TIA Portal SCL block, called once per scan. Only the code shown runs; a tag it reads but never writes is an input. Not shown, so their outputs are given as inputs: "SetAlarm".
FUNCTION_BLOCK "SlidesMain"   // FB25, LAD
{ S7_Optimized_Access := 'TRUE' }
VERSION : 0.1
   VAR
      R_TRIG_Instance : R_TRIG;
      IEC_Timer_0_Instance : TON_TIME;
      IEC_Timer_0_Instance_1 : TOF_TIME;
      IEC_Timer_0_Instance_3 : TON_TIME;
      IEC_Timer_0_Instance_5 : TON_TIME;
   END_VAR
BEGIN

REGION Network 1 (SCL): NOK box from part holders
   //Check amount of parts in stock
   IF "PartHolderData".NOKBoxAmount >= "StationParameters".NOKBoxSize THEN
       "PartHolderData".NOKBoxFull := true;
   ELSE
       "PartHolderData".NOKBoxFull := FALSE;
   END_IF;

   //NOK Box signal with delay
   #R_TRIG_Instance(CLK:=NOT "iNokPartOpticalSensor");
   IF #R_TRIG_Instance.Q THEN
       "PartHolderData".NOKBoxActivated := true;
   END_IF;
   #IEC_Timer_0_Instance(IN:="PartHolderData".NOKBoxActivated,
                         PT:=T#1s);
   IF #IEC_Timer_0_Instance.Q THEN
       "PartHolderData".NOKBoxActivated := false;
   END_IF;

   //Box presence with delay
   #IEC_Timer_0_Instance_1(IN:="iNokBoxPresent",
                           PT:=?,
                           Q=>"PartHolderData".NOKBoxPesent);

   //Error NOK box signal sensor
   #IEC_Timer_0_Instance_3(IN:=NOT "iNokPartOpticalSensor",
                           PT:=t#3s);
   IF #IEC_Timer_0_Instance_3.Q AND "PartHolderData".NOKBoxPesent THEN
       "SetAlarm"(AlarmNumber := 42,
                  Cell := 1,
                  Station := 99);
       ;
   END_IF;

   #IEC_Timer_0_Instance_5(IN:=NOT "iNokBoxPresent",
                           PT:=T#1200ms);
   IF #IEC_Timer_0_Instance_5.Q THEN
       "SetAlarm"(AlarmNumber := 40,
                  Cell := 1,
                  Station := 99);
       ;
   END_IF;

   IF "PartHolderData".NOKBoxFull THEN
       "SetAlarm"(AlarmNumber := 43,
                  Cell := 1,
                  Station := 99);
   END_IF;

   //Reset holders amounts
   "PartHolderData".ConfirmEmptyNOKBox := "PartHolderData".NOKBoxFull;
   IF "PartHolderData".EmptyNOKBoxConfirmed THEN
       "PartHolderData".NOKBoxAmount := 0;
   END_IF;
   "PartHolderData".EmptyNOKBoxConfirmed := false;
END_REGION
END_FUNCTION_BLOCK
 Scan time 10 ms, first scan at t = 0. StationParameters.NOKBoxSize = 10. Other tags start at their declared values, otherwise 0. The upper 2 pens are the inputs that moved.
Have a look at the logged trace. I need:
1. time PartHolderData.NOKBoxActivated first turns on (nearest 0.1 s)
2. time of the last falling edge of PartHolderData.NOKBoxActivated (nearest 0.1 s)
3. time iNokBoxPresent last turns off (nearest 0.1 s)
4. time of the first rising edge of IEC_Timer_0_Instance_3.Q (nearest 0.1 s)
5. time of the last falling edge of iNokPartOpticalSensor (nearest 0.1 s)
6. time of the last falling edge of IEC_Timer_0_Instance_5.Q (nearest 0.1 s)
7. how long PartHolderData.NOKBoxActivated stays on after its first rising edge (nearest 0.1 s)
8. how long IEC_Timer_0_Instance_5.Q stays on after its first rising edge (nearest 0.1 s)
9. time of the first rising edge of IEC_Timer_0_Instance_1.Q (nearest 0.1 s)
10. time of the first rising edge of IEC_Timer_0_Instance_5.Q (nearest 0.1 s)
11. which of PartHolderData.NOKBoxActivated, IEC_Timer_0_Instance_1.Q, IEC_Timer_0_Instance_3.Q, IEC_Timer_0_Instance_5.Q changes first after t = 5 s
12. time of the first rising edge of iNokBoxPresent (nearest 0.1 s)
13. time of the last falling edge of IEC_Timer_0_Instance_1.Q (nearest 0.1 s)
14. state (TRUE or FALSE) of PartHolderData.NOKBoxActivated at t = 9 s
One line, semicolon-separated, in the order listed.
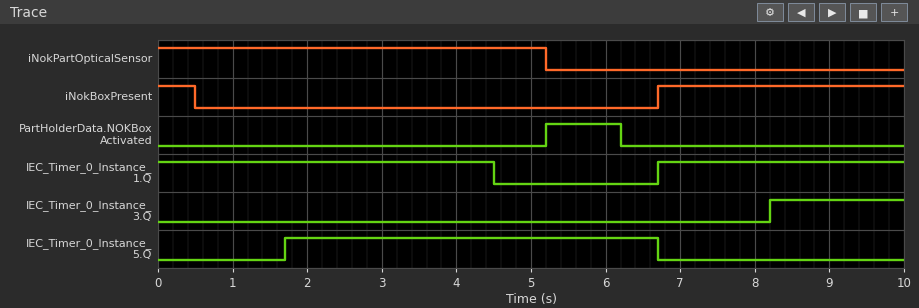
5.2 s; 6.2 s; 0.5 s; 8.2 s; 5.2 s; 6.7 s; 1.0 s; 5.0 s; 6.7 s; 1.7 s; PartHolderData.NOKBoxActivated; 6.7 s; 4.5 s; FALSE
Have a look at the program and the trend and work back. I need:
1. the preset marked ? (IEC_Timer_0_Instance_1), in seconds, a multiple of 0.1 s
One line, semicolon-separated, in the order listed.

4.0 s
